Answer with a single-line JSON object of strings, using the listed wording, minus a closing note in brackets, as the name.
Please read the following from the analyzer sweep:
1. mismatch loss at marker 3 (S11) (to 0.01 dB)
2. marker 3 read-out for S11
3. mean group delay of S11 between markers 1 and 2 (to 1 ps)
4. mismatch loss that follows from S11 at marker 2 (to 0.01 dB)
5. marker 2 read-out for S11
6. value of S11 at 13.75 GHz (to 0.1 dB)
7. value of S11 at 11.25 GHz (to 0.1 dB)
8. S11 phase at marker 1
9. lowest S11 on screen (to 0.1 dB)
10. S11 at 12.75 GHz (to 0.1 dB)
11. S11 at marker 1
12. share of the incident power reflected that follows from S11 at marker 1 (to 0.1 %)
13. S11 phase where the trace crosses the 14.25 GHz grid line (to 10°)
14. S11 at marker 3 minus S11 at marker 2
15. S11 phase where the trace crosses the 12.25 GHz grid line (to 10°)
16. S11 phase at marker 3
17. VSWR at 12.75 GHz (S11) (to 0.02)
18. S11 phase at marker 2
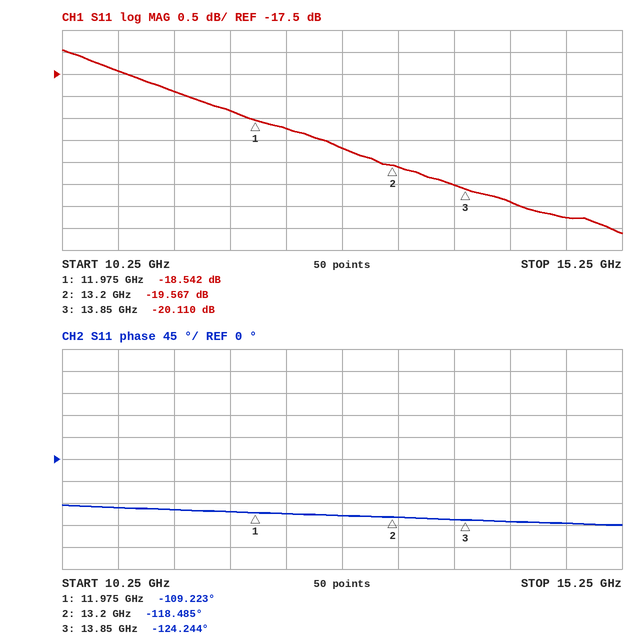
{"mismatch loss at marker 3 (S11)": "0.04 dB", "marker 3 read-out for S11": "-20.110 dB", "mean group delay of S11 between markers 1 and 2": "21 ps", "mismatch loss that follows from S11 at marker 2": "0.05 dB", "marker 2 read-out for S11": "-19.567 dB", "value of S11 at 13.75 GHz": "-20.0 dB", "value of S11 at 11.25 GHz": "-17.9 dB", "S11 phase at marker 1": "-109.223°", "lowest S11 on screen": "-21.1 dB", "S11 at 12.75 GHz": "-19.2 dB", "S11 at marker 1": "-18.542 dB", "share of the incident power reflected that follows from S11 at marker 1": "1.4 %", "S11 phase where the trace crosses the 14.25 GHz grid line": "-130°", "S11 at marker 3 minus S11 at marker 2": "-0.543 dB", "S11 phase where the trace crosses the 12.25 GHz grid line": "-110°", "S11 phase at marker 3": "-124.244°", "VSWR at 12.75 GHz (S11)": "1.24", "S11 phase at marker 2": "-118.485°"}
